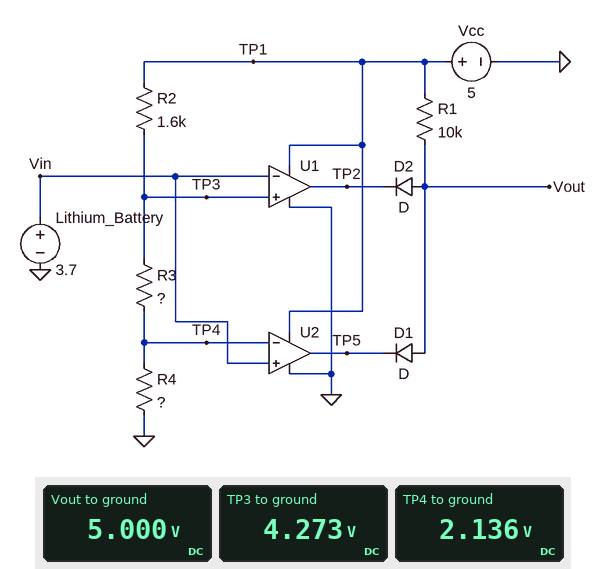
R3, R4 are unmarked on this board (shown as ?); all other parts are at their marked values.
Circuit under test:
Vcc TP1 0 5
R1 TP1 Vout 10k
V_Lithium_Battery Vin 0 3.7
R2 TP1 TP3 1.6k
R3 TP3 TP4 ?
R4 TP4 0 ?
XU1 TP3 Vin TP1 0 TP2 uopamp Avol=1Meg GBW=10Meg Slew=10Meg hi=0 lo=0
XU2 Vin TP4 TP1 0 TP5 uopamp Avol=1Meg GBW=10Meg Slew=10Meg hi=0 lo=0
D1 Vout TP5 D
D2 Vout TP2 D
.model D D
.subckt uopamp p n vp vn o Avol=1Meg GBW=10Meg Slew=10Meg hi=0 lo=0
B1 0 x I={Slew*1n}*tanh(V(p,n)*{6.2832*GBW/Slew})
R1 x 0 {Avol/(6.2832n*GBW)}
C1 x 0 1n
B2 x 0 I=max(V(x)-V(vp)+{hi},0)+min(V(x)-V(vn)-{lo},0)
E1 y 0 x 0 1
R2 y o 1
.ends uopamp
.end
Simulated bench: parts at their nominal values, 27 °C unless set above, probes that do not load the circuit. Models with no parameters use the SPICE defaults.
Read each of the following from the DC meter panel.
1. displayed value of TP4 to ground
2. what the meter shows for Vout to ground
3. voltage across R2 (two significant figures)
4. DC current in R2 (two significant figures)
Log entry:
2.136 V
5.000 V
730 mV
450 µA
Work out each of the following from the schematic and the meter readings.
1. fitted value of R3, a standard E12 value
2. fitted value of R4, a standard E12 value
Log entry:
4.7 kΩ
4.7 kΩ
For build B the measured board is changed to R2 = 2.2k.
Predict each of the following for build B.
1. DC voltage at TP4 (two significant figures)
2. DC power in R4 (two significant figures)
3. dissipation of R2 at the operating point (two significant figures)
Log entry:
2.0 V
870 µW
410 µW
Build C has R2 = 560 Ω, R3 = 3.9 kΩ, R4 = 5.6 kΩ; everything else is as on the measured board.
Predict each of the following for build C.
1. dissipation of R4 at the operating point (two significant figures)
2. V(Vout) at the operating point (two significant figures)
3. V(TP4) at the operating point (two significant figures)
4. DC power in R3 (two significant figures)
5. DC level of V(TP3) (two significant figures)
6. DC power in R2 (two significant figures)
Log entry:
1.4 mW
5.0 V
2.8 V
960 µW
4.7 V
140 µW
